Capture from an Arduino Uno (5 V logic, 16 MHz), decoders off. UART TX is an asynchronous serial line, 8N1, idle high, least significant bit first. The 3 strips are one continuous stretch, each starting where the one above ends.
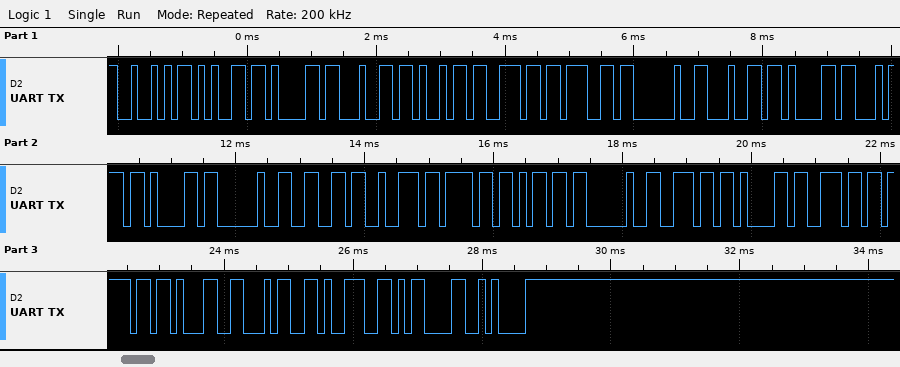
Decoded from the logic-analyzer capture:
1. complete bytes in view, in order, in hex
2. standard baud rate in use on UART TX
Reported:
52 65 61 64 69 6E 67 20 64 61 74 61 20 66 72 6F 6D 20 6E 61 6E 6F 31 34 39 0D 0A
9600 baud
